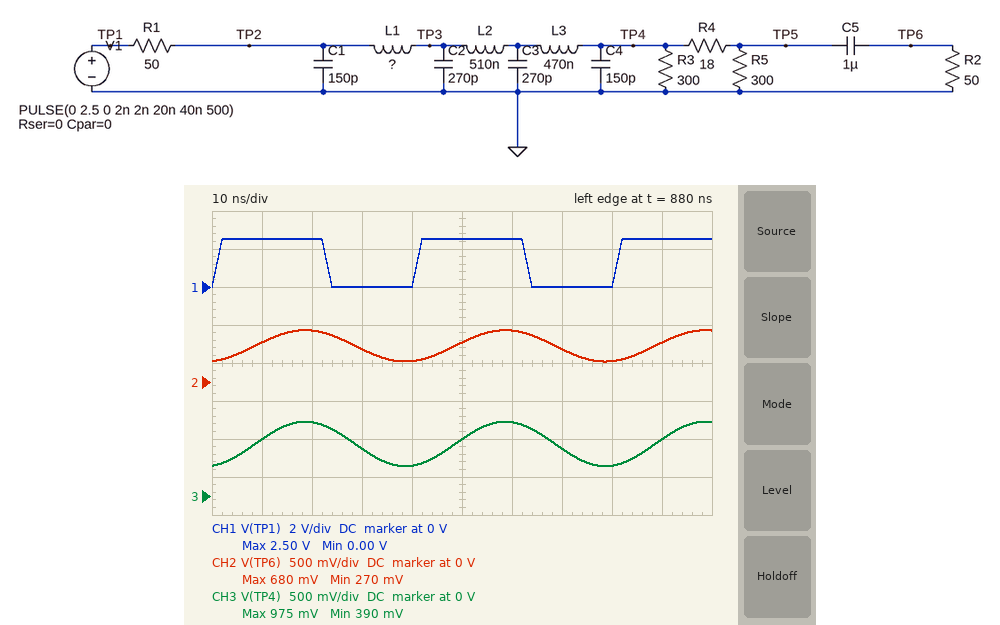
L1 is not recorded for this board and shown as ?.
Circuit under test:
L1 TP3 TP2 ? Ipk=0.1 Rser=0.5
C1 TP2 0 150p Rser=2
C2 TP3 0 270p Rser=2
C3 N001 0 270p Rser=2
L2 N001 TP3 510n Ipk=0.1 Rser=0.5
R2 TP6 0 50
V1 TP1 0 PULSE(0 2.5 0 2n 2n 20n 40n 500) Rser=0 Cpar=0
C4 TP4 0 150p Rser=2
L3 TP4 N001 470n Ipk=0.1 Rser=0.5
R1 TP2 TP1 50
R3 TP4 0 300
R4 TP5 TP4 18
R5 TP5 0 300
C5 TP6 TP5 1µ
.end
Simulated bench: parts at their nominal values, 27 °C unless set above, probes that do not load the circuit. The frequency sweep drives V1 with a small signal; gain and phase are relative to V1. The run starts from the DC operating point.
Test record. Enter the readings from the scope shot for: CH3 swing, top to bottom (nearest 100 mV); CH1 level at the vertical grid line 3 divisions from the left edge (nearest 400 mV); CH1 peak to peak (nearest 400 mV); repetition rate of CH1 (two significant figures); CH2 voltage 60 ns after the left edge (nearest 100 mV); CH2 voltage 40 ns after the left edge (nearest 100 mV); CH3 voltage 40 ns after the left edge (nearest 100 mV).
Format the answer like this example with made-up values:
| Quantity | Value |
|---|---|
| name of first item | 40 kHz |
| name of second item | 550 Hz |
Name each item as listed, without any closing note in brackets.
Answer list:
| Quantity | Value |
|---|---|
| CH3 swing, top to bottom | 600 mV |
| CH1 level at the vertical grid line 3 divisions from the left edge | 0 V |
| CH1 peak to peak | 2.4 V |
| repetition rate of CH1 | 25 MHz |
| CH2 voltage 60 ns after the left edge | 700 mV |
| CH2 voltage 40 ns after the left edge | 300 mV |
| CH3 voltage 40 ns after the left edge | 400 mV |
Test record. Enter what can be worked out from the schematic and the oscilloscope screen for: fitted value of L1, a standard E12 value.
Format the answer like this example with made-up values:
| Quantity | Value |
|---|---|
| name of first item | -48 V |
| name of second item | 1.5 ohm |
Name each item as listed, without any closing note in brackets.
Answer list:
| Quantity | Value |
|---|---|
| fitted value of L1, a standard E12 value | 680 nH |
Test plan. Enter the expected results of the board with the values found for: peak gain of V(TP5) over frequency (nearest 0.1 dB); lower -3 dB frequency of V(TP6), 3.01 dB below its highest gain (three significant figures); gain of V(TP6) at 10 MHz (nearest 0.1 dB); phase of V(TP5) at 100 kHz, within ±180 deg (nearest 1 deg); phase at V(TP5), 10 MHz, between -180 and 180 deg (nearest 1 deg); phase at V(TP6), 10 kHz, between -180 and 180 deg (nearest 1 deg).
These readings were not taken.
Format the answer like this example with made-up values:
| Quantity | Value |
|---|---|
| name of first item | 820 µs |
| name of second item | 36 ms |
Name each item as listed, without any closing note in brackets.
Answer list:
| Quantity | Value |
|---|---|
| peak gain of V(TP5) over frequency | -3.0 dB |
| lower -3 dB frequency of V(TP6), 3.01 dB below its highest gain | 1.57 kHz |
| gain of V(TP6) at 10 MHz | -9.6 dB |
| phase of V(TP5) at 100 kHz, within ±180 deg | -2 deg |
| phase at V(TP5), 10 MHz, between -180 and 180 deg | -138 deg |
| phase at V(TP6), 10 kHz, between -180 and 180 deg | 9 deg |
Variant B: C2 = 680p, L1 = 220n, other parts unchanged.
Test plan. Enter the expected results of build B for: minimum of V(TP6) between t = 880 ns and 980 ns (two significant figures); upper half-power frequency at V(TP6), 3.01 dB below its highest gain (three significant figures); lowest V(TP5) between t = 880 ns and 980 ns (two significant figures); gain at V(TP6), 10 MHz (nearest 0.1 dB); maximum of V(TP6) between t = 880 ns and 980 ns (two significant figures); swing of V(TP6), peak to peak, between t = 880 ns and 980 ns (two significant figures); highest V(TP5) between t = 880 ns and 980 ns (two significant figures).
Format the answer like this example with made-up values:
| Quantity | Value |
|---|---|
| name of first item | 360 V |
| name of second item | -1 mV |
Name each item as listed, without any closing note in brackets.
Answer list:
| Quantity | Value |
|---|---|
| minimum of V(TP6) between t = 880 ns and 980 ns | 340 mV |
| upper half-power frequency at V(TP6), 3.01 dB below its highest gain | 11.3 MHz |
| lowest V(TP5) between t = 880 ns and 980 ns | 350 mV |
| gain at V(TP6), 10 MHz | -11.7 dB |
| maximum of V(TP6) between t = 880 ns and 980 ns | 610 mV |
| swing of V(TP6), peak to peak, between t = 880 ns and 980 ns | 270 mV |
| highest V(TP5) between t = 880 ns and 980 ns | 620 mV |
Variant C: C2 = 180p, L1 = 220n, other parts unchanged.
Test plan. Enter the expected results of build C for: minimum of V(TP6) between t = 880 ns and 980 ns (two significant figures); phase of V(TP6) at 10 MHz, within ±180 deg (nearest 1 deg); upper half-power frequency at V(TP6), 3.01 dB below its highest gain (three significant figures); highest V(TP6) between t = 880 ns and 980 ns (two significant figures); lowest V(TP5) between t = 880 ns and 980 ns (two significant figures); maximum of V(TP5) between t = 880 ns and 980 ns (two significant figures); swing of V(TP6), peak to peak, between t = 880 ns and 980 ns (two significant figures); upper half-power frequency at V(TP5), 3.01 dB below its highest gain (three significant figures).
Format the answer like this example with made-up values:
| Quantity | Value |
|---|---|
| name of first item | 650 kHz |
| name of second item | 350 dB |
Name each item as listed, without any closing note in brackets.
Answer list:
| Quantity | Value |
|---|---|
| minimum of V(TP6) between t = 880 ns and 980 ns | 200 mV |
| phase of V(TP6) at 10 MHz, within ±180 deg | -111 deg |
| upper half-power frequency at V(TP6), 3.01 dB below its highest gain | 22.2 MHz |
| highest V(TP6) between t = 880 ns and 980 ns | 750 mV |
| lowest V(TP5) between t = 880 ns and 980 ns | 210 mV |
| maximum of V(TP5) between t = 880 ns and 980 ns | 760 mV |
| swing of V(TP6), peak to peak, between t = 880 ns and 980 ns | 550 mV |
| upper half-power frequency at V(TP5), 3.01 dB below its highest gain | 2.19 kHz |
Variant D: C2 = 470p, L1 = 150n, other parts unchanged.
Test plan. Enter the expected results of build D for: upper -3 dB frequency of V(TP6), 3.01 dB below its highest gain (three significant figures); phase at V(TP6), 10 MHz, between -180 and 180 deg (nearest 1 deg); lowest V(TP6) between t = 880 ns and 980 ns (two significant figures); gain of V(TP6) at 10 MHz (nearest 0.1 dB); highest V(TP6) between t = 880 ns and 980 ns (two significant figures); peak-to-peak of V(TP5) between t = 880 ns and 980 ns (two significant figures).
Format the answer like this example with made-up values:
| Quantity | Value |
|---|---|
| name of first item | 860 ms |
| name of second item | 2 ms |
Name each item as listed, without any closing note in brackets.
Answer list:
| Quantity | Value |
|---|---|
| upper -3 dB frequency of V(TP6), 3.01 dB below its highest gain | 14.0 MHz |
| phase at V(TP6), 10 MHz, between -180 and 180 deg | -127 deg |
| lowest V(TP6) between t = 880 ns and 980 ns | 310 mV |
| gain of V(TP6) at 10 MHz | -10.7 dB |
| highest V(TP6) between t = 880 ns and 980 ns | 650 mV |
| peak-to-peak of V(TP5) between t = 880 ns and 980 ns | 340 mV |
